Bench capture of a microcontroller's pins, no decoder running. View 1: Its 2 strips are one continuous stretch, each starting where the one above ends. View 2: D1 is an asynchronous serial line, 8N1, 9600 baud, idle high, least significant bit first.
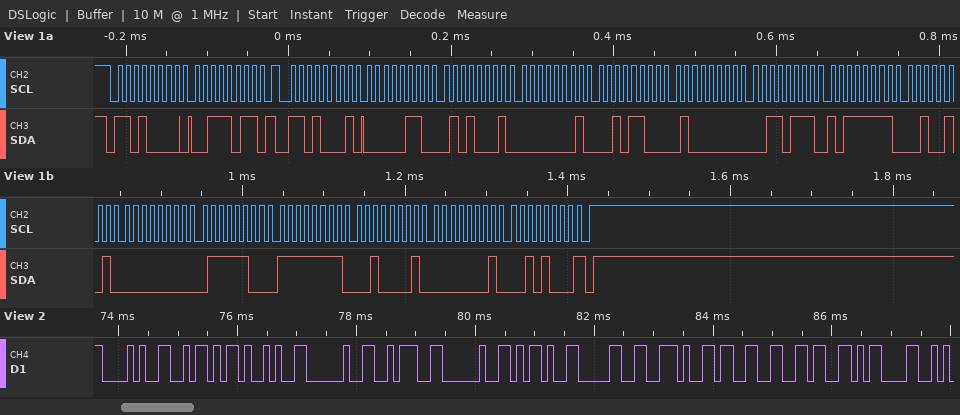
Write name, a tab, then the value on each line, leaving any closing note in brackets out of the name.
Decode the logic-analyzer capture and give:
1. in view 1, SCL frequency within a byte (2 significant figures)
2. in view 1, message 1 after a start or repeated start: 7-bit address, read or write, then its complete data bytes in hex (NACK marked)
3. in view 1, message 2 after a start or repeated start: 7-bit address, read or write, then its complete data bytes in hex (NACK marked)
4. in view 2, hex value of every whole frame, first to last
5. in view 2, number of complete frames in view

in view 1, SCL frequency within a byte	100 kHz
in view 1, message 1 after a start or repeated start: 7-bit address, read or write, then its complete data bytes in hex	0x68 write: 3B
in view 1, message 2 after a start or repeated start: 7-bit address, read or write, then its complete data bytes in hex	0x68 read: 06 51 01 2C 40 37 BF 25 00 7C FF 21 01 28 NACK
in view 2, hex value of every whole frame, first to last	28 5A 29 20 3A 20 2D 30 2E 33 36 0D
in view 2, number of complete frames in view	12
